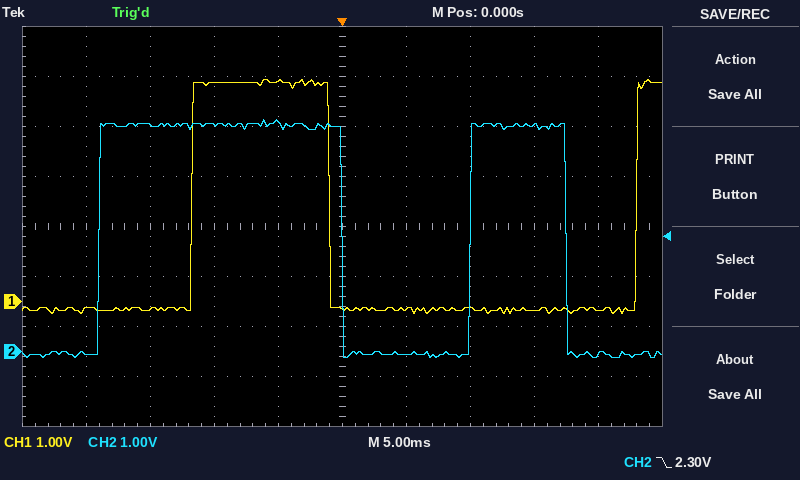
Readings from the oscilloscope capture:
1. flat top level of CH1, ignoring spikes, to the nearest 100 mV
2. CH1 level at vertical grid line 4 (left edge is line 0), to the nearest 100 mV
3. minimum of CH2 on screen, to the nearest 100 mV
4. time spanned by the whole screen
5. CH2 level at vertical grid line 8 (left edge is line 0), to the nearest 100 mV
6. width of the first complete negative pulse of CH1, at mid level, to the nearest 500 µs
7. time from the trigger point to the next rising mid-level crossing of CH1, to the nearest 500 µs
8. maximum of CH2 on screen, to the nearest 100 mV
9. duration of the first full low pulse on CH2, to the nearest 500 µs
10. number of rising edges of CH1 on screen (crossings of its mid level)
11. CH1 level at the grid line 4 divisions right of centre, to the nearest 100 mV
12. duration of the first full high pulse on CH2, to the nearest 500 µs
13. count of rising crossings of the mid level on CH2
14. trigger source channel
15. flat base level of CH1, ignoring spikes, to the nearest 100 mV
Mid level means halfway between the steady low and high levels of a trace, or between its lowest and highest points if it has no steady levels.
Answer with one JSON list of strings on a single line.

["4.4 V", "4.4 V", "-100 mV", "50 ms", "4.5 V", "24.0 ms", "23.0 ms", "4.6 V", "10.0 ms", "2", "-200 mV", "19.0 ms", "2", "CH2", "-200 mV"]
